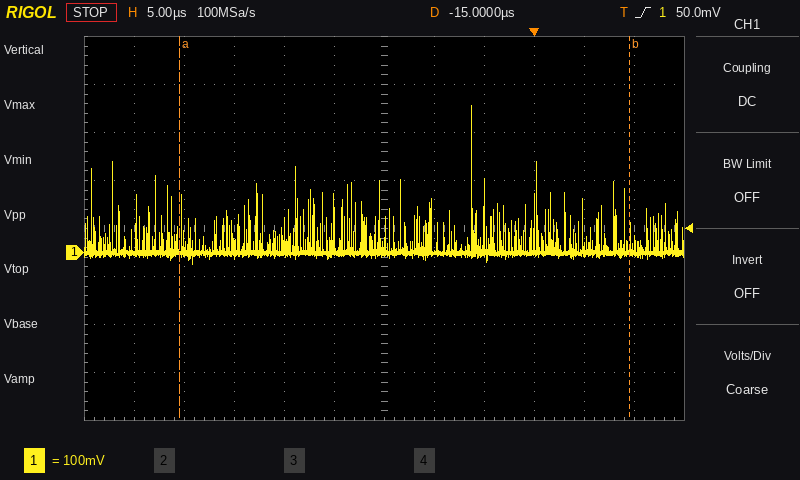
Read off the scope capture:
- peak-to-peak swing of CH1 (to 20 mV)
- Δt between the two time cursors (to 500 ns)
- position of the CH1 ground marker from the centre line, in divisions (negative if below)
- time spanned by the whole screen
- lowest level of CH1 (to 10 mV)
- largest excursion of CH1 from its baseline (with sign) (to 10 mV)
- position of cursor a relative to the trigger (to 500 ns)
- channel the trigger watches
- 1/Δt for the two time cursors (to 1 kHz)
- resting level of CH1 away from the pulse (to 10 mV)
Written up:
320 mV
45.0 µs
-0.5 div
60 µs
-20 mV
+300 mV
-35.5 µs
CH1
22 kHz
0 mV
